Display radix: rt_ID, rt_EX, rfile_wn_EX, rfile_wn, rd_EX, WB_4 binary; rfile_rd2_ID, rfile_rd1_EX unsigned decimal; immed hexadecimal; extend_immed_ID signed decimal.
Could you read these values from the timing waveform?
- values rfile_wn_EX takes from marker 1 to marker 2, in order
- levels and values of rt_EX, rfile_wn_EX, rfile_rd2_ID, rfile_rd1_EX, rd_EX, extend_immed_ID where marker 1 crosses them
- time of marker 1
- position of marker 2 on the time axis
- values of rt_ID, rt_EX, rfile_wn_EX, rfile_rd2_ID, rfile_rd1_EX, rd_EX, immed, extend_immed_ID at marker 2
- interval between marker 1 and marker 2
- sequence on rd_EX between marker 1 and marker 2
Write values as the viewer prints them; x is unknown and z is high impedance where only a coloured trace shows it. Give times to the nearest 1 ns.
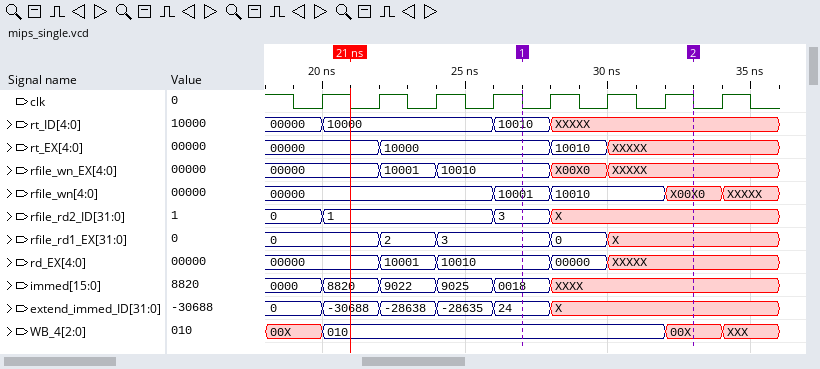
10010, X00X0, XXXXX
rt_EX=10000, rfile_wn_EX=10010, rfile_rd2_ID=3, rfile_rd1_EX=3, rd_EX=10010, extend_immed_ID=24
27 ns
33 ns
rt_ID=XXXXX, rt_EX=XXXXX, rfile_wn_EX=XXXXX, rfile_rd2_ID=X, rfile_rd1_EX=X, rd_EX=XXXXX, immed=XXXX, extend_immed_ID=X
6 ns
10010, 00000, XXXXX
